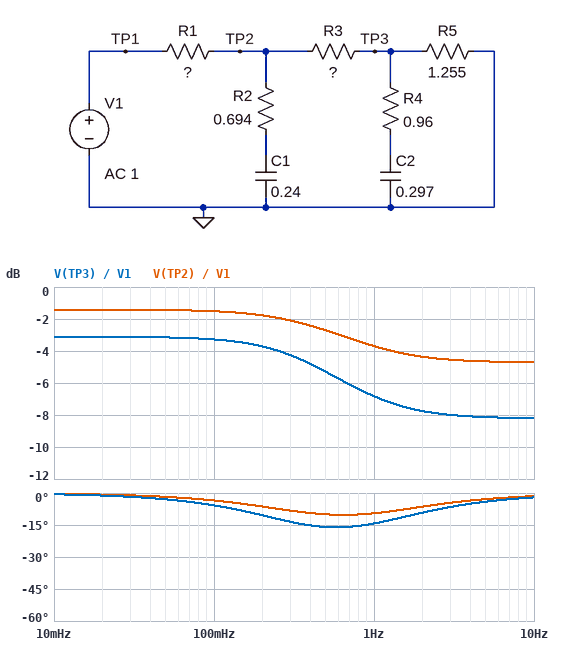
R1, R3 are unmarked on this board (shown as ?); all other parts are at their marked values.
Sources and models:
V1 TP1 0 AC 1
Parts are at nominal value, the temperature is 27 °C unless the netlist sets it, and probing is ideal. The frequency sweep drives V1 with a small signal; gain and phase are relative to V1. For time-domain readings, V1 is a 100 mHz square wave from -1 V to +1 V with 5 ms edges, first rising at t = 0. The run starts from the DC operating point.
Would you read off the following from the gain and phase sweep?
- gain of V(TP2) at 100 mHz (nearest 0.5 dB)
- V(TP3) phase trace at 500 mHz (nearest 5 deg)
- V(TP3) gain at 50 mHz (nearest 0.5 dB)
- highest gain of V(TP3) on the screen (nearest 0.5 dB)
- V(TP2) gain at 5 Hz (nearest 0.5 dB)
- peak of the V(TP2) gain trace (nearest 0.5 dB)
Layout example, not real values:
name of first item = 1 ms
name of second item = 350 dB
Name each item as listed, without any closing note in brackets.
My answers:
gain of V(TP2) at 100 mHz = -1.5 dB
V(TP3) phase trace at 500 mHz = -15 deg
V(TP3) gain at 50 mHz = -3.0 dB
highest gain of V(TP3) on the screen = -3.0 dB
V(TP2) gain at 5 Hz = -4.5 dB
peak of the V(TP2) gain trace = -1.5 dB
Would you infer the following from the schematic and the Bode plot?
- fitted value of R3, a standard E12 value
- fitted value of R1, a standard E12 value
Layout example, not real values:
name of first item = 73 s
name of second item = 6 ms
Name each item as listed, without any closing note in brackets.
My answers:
fitted value of R3, a standard E12 value = 0.27 Ω
fitted value of R1, a standard E12 value = 0.27 Ω
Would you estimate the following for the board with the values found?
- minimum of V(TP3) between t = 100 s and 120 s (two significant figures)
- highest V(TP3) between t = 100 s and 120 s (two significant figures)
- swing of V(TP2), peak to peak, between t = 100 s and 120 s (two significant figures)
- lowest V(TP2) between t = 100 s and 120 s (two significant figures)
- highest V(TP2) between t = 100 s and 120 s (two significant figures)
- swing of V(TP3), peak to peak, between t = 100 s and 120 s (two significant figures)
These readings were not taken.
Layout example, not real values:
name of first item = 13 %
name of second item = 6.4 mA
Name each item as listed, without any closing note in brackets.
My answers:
minimum of V(TP3) between t = 100 s and 120 s = -700 mV
highest V(TP3) between t = 100 s and 120 s = 700 mV
swing of V(TP2), peak to peak, between t = 100 s and 120 s = 1.7 V
lowest V(TP2) between t = 100 s and 120 s = -850 mV
highest V(TP2) between t = 100 s and 120 s = 850 mV
swing of V(TP3), peak to peak, between t = 100 s and 120 s = 1.4 V
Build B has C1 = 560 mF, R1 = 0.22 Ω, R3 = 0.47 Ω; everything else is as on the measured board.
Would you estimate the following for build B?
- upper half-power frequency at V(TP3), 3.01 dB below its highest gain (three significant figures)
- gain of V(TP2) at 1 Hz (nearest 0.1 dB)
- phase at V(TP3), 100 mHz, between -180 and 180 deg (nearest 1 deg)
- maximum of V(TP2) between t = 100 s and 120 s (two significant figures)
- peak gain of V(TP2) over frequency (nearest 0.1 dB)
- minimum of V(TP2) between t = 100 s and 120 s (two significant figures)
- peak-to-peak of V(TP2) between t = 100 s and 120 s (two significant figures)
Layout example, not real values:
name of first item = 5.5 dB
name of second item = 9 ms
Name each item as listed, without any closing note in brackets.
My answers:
upper half-power frequency at V(TP3), 3.01 dB below its highest gain = 470 mHz
gain of V(TP2) at 1 Hz = -3.4 dB
phase at V(TP3), 100 mHz, between -180 and 180 deg = -8 deg
maximum of V(TP2) between t = 100 s and 120 s = 890 mV
peak gain of V(TP2) over frequency = -1.0 dB
minimum of V(TP2) between t = 100 s and 120 s = -890 mV
peak-to-peak of V(TP2) between t = 100 s and 120 s = 1.8 V
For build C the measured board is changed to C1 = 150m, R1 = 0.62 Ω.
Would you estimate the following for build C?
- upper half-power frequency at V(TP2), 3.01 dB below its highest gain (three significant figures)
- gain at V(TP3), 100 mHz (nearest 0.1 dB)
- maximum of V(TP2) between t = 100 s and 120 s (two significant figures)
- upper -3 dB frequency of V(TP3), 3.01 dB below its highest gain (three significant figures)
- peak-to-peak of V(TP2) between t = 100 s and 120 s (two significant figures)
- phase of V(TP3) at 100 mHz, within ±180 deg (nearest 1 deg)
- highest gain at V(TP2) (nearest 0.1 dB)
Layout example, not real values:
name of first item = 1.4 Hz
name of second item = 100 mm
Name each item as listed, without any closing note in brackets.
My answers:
upper half-power frequency at V(TP2), 3.01 dB below its highest gain = 894 mHz
gain at V(TP3), 100 mHz = -4.9 dB
maximum of V(TP2) between t = 100 s and 120 s = 710 mV
upper -3 dB frequency of V(TP3), 3.01 dB below its highest gain = 546 mHz
peak-to-peak of V(TP2) between t = 100 s and 120 s = 1.4 V
phase of V(TP3) at 100 mHz, within ±180 deg = -8 deg
highest gain at V(TP2) = -3.0 dB
